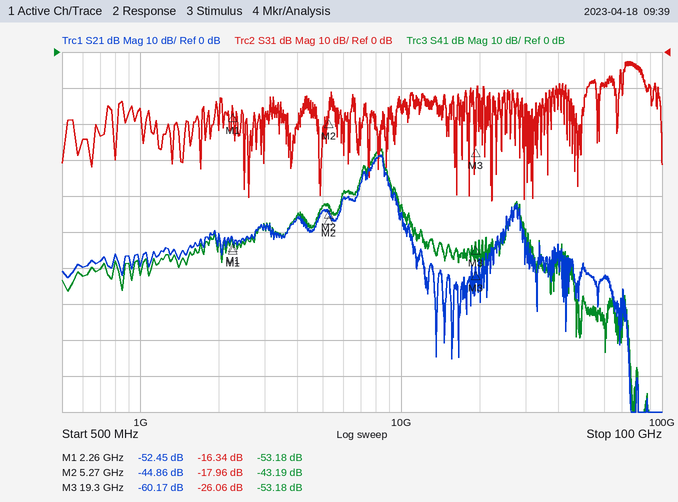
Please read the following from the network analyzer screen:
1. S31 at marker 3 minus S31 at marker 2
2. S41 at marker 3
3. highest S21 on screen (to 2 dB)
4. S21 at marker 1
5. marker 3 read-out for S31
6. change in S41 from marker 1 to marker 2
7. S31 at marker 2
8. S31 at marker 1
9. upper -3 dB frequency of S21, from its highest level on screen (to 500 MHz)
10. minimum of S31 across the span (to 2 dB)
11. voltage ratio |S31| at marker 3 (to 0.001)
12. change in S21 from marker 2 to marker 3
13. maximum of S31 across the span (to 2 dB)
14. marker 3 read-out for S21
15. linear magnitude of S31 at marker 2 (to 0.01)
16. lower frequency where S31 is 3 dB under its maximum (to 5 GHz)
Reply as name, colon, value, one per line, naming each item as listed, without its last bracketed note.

S31 at marker 3 minus S31 at marker 2: -8.10 dB
S41 at marker 3: -53.18 dB
highest S21 on screen: -28 dB
S21 at marker 1: -52.45 dB
marker 3 read-out for S31: -26.06 dB
change in S41 from marker 1 to marker 2: 9.99 dB
S31 at marker 2: -17.96 dB
S31 at marker 1: -16.34 dB
upper -3 dB frequency of S21, from its highest level on screen: 8.5 GHz
minimum of S31 across the span: -42 dB
voltage ratio |S31| at marker 3: 0.050
change in S21 from marker 2 to marker 3: -15.31 dB
maximum of S31 across the span: -2 dB
marker 3 read-out for S21: -60.17 dB
linear magnitude of S31 at marker 2: 0.13
lower frequency where S31 is 3 dB under its maximum: 70 GHz
